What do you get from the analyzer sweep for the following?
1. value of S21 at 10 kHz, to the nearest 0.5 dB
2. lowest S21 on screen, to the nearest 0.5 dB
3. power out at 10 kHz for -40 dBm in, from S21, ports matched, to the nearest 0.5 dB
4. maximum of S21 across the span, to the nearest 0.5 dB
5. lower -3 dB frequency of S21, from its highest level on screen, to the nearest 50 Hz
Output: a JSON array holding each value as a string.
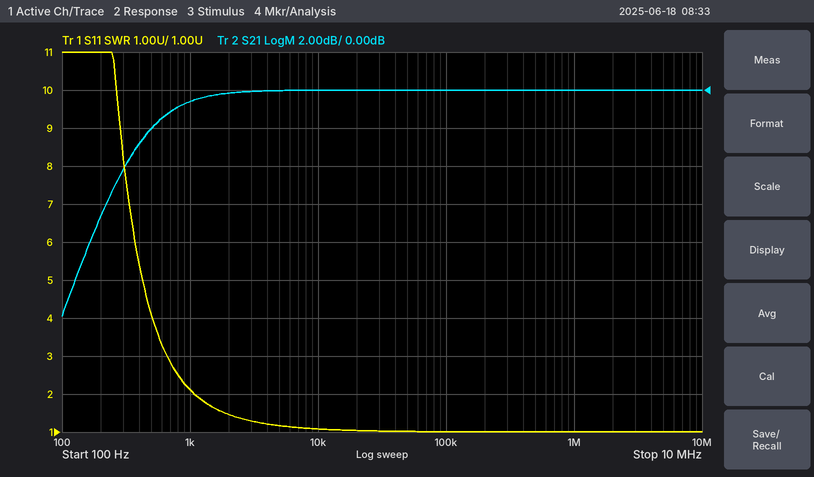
["0.0 dB", "-12.0 dB", "-40.0 dBm", "0.0 dB", "400 Hz"]
